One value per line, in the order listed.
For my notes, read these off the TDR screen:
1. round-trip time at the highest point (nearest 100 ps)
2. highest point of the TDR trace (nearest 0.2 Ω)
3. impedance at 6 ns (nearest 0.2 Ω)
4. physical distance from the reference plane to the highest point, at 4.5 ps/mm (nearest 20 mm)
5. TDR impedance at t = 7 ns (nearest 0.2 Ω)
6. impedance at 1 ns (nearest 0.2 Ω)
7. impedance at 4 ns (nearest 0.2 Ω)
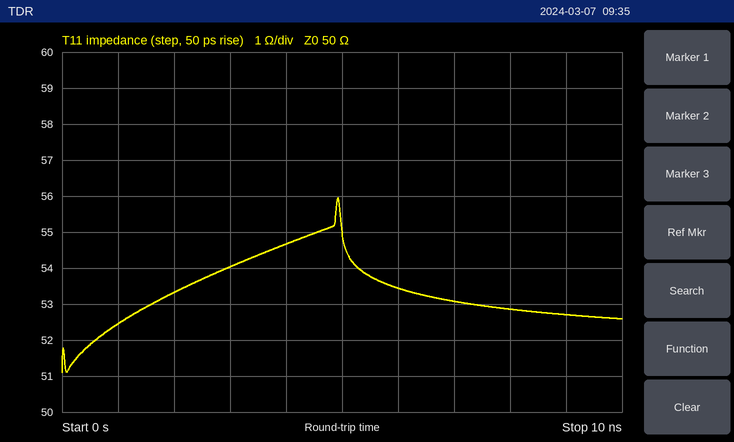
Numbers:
4.9 ns
56.0 Ω
53.4 Ω
540 mm
53.0 Ω
52.4 Ω
54.6 Ω
